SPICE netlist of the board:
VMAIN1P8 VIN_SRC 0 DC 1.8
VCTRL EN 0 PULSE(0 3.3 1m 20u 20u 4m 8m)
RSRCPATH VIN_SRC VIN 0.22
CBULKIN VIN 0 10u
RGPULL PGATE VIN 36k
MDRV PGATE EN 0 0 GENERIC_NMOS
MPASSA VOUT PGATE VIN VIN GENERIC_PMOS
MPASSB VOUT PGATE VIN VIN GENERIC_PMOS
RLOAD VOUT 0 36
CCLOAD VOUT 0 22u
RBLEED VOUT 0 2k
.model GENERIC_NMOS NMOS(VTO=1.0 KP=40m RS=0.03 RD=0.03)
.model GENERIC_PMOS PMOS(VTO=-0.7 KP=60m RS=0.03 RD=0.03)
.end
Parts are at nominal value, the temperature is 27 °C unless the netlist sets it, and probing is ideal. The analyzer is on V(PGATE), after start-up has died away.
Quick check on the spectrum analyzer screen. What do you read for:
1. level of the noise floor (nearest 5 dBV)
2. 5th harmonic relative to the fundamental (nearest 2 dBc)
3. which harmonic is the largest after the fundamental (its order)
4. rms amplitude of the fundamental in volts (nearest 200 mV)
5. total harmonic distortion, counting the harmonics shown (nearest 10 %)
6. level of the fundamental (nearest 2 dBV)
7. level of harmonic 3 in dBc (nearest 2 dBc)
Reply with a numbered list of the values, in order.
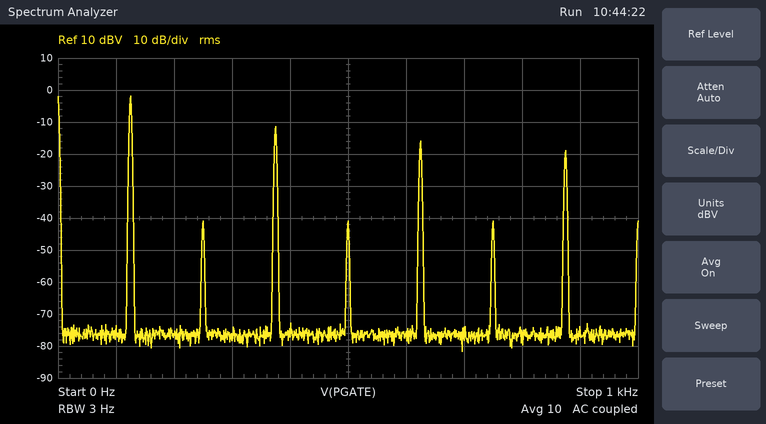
1. -75 dBV
2. -14 dBc
3. 3
4. 800 mV
5. 40 %
6. -2 dBV
7. -10 dBc
